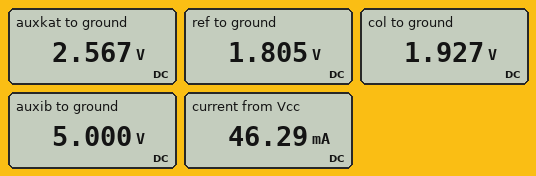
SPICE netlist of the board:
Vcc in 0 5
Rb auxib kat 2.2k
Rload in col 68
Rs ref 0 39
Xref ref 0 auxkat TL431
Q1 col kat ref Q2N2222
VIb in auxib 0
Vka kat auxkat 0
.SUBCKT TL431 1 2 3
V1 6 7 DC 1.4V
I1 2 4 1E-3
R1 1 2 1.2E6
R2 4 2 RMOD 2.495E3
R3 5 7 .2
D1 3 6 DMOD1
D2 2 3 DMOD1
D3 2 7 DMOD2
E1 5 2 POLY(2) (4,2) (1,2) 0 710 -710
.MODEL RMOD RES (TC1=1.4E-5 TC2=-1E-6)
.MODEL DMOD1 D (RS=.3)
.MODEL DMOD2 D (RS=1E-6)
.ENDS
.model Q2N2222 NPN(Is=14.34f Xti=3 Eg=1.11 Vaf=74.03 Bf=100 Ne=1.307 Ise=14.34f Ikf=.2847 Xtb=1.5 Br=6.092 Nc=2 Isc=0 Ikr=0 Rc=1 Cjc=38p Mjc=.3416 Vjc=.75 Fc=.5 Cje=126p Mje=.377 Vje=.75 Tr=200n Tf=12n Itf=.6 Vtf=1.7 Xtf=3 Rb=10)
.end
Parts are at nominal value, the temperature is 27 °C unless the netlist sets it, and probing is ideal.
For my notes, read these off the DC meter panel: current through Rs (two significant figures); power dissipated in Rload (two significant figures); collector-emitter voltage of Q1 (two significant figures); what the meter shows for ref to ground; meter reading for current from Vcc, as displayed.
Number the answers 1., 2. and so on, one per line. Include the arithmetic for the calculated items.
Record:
1. (1.805 V) / 39 Ω = 46 mA
2. (5 V - 1.927 V)^2 / 68 Ω = 140 mW
3. 1.927 V - 1.805 V = 120 mV
4. 1.805 V
5. 46.29 mA
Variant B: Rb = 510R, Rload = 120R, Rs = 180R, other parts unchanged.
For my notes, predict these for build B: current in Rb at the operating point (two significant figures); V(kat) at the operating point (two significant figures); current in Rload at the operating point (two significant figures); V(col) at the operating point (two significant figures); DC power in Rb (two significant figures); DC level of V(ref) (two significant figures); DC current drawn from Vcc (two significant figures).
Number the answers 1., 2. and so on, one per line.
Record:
1. 3.5 mA
2. 3.2 V
3. 14 mA
4. 3.4 V
5. 6.3 mW
6. 2.5 V
7. 17 mA
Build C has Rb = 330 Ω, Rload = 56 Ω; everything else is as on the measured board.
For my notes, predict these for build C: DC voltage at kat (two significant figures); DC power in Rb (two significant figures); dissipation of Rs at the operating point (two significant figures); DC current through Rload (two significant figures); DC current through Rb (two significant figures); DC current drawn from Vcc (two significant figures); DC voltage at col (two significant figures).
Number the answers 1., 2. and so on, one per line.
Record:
1. 3.0 V
2. 12 mW
3. 120 mW
4. 49 mA
5. 6.1 mA
6. 55 mA
7. 2.2 V
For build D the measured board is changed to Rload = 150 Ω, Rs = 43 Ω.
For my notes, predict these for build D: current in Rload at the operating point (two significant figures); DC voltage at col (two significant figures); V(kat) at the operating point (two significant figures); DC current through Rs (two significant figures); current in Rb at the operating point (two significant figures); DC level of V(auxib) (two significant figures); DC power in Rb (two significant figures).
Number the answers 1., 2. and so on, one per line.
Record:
1. 25 mA
2. 1.2 V
3. 1.9 V
4. 27 mA
5. 1.4 mA
6. 5.0 V
7. 4.4 mW
